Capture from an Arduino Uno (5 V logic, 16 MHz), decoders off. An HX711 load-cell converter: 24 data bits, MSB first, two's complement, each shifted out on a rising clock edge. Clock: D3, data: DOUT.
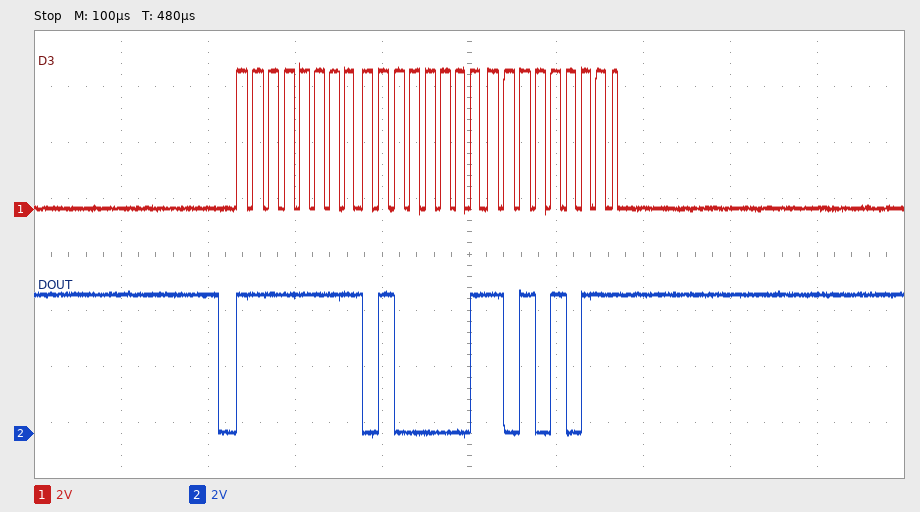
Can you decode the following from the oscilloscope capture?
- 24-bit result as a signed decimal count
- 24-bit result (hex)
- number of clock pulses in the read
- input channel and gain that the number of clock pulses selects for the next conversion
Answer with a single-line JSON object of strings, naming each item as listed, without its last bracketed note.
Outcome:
{"24-bit result as a signed decimal count": "-48725", "24-bit result": "0xFF41AB", "number of clock pulses in the read": "25", "input channel and gain that the number of clock pulses selects for the next conversion": "channel A, gain 128"}
